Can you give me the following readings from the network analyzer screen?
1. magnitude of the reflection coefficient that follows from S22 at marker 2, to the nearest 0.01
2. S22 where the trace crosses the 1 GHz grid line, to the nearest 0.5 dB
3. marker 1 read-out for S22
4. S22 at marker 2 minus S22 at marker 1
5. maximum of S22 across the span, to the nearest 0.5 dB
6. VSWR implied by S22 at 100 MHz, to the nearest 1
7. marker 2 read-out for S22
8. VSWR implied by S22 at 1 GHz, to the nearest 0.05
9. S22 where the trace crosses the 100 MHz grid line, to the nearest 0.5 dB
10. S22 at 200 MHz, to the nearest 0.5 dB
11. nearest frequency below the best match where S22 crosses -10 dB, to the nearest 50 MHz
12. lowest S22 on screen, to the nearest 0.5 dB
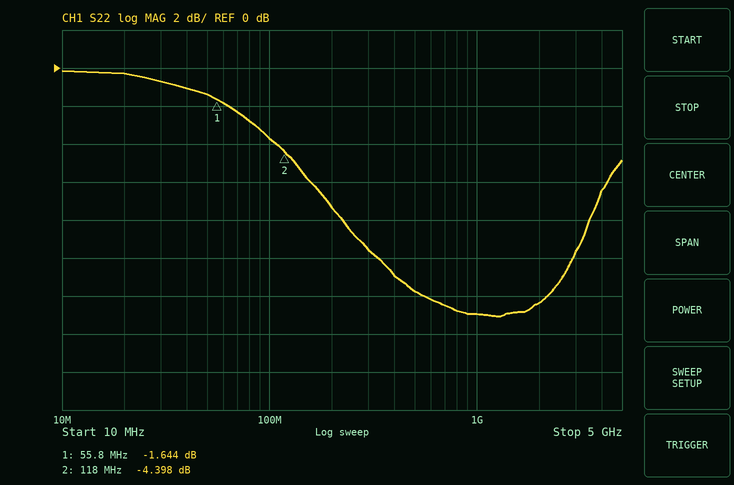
0.60
-13.0 dB
-1.644 dB
-2.754 dB
0.0 dB
5
-4.398 dB
1.60
-3.5 dB
-7.5 dB
350 MHz
-13.0 dB
